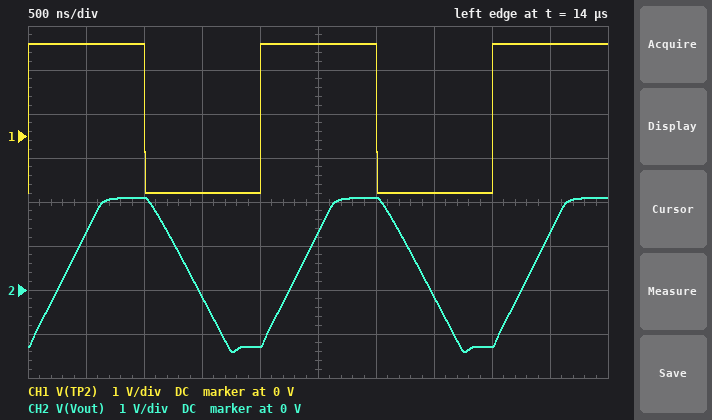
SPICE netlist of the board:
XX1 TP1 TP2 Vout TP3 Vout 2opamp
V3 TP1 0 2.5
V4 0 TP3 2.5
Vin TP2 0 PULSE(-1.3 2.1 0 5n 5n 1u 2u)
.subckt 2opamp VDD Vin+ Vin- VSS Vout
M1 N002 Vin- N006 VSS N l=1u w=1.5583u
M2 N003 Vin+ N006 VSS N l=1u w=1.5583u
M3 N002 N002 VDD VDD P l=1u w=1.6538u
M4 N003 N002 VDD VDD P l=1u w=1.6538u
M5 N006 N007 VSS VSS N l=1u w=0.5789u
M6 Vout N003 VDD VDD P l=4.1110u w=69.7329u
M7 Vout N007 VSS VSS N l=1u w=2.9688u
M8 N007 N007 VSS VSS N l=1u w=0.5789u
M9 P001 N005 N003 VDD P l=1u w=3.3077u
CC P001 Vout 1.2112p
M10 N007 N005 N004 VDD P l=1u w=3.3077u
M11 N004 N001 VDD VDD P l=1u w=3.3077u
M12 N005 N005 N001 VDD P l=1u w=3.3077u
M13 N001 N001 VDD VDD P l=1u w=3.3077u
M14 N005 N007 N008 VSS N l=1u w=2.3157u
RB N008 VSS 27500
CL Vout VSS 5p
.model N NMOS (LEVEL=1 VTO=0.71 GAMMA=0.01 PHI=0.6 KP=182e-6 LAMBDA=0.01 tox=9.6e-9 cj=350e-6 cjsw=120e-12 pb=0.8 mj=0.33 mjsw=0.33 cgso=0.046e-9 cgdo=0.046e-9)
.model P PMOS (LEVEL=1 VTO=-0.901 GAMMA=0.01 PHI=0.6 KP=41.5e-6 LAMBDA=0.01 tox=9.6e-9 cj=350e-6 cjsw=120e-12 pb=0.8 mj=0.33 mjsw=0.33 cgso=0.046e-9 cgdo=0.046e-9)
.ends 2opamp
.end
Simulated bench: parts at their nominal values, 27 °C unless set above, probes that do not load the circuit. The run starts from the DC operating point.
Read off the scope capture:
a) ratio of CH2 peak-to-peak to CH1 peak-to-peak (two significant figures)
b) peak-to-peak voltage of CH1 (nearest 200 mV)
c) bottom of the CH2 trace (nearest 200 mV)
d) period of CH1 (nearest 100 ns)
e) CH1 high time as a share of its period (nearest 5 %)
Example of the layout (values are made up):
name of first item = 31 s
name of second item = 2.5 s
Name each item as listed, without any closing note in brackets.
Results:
ratio of CH2 peak-to-peak to CH1 peak-to-peak = 1.0
peak-to-peak voltage of CH1 = 3.4 V
bottom of the CH2 trace = -1.4 V
period of CH1 = 2.0 µs
CH1 high time as a share of its period = 50 %
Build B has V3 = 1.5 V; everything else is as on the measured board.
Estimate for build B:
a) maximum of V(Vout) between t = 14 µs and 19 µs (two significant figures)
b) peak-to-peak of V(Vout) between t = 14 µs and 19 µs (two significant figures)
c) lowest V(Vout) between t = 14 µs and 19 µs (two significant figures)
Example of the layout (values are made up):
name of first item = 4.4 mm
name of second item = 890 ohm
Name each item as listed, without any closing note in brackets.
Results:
maximum of V(Vout) between t = 14 µs and 19 µs = 1.3 V
peak-to-peak of V(Vout) between t = 14 µs and 19 µs = 2.7 V
lowest V(Vout) between t = 14 µs and 19 µs = -1.4 V
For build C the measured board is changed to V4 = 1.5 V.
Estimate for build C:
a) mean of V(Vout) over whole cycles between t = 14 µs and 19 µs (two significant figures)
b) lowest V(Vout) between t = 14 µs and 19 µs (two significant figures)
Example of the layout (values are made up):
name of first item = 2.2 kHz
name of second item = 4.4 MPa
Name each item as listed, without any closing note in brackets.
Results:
mean of V(Vout) over whole cycles between t = 14 µs and 19 µs = 700 mV
lowest V(Vout) between t = 14 µs and 19 µs = -850 mV
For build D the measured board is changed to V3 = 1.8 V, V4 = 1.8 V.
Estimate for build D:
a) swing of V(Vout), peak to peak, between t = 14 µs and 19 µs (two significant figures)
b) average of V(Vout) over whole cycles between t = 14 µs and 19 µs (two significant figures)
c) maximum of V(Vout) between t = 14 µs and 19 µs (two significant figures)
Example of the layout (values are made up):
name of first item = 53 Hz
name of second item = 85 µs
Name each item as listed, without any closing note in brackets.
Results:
swing of V(Vout), peak to peak, between t = 14 µs and 19 µs = 2.7 V
average of V(Vout) over whole cycles between t = 14 µs and 19 µs = 290 mV
maximum of V(Vout) between t = 14 µs and 19 µs = 1.6 V
